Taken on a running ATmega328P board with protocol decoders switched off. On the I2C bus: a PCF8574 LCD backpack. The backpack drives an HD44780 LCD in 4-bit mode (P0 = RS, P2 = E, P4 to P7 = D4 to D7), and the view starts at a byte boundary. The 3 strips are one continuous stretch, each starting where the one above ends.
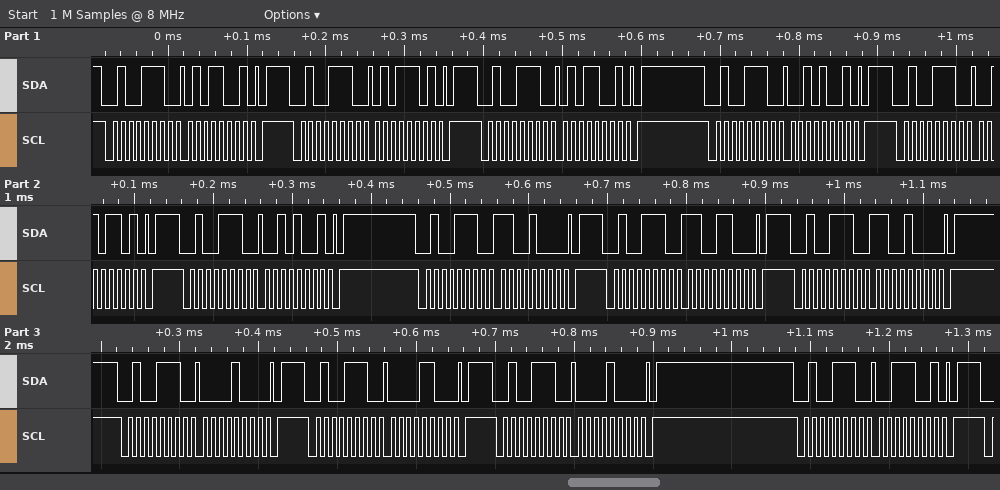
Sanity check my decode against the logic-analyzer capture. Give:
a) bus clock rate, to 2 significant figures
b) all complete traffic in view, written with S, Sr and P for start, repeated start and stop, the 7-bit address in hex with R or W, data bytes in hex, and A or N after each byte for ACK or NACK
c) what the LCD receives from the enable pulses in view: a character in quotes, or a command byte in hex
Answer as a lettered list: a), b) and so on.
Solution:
a) 100 kHz
b) S 27W A 59 A P S 27W A 5D A P S 27W A 59 A P S 27W A 29 A P S 27W A 2D A P S 27W A 29 A P S 27W A C8 A P S 27W A CC A P S 27W A C8 A P S 27W A 08 A P S 27W A 0C A P S 27W A 08 A P S 27W A 39 A P
c) 'R' 0xC0
